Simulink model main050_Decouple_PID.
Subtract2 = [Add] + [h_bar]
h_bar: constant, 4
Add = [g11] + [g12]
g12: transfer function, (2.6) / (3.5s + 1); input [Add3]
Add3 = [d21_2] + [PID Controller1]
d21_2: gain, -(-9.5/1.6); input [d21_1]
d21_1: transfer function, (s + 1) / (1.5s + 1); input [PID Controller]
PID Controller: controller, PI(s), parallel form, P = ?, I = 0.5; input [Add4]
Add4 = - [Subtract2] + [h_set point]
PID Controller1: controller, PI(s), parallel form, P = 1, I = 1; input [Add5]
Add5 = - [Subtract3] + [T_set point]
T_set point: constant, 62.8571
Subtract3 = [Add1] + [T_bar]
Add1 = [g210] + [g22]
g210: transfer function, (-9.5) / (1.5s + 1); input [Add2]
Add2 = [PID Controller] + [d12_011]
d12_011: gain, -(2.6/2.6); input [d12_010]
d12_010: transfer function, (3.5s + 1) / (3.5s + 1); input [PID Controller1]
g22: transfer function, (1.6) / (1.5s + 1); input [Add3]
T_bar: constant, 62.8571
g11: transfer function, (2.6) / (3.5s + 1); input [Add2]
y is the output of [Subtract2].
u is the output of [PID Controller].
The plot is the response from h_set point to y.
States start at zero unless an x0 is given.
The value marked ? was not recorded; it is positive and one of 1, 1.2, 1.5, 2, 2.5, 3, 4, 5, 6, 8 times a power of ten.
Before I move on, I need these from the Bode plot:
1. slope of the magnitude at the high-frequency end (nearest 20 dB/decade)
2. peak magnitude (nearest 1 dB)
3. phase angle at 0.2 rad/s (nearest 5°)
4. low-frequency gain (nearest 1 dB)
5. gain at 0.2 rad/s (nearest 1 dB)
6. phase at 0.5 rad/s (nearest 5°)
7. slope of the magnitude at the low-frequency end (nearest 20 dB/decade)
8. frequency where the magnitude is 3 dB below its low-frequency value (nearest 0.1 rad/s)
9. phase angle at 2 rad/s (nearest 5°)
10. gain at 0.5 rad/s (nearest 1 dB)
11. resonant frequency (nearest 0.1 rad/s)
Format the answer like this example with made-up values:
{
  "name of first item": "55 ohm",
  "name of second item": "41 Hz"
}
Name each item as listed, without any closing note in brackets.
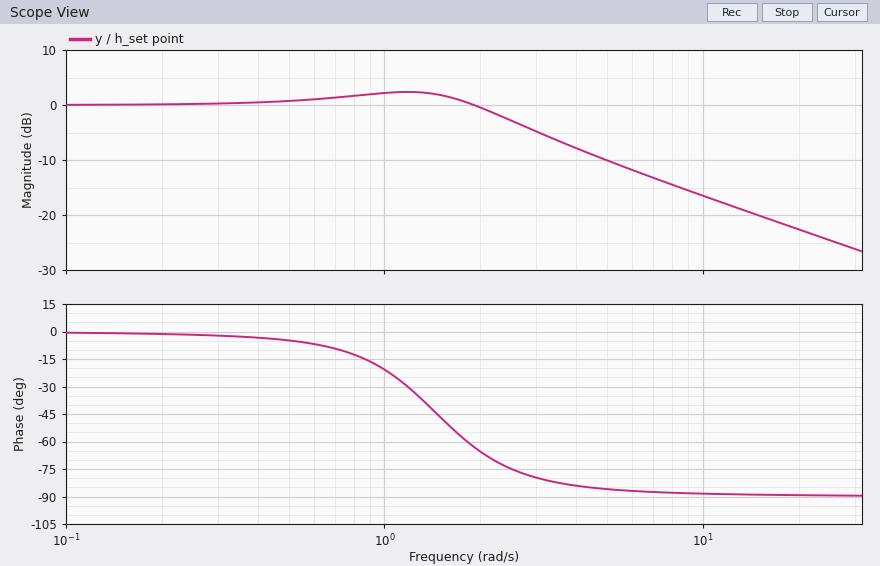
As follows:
{
  "slope of the magnitude at the high-frequency end": "-20 dB/decade",
  "peak magnitude": "2 dB",
  "phase angle at 0.2 rad/s": "0°",
  "low-frequency gain": "0 dB",
  "gain at 0.2 rad/s": "0 dB",
  "phase at 0.5 rad/s": "-5°",
  "slope of the magnitude at the low-frequency end": "0 dB/decade",
  "frequency where the magnitude is 3 dB below its low-frequency value": "2.5 rad/s",
  "phase angle at 2 rad/s": "-65°",
  "gain at 0.5 rad/s": "1 dB",
  "resonant frequency": "1.2 rad/s"
}
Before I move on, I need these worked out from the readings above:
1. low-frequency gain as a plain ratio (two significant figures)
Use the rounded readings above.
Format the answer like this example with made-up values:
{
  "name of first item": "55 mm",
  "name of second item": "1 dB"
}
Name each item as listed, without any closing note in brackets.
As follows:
{
  "low-frequency gain as a plain ratio": "1.0"
}
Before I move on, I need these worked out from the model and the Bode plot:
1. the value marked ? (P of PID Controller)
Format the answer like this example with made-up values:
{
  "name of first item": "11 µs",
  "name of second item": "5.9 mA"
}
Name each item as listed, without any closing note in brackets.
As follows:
{
  "the value marked ?": "0.4"
}
